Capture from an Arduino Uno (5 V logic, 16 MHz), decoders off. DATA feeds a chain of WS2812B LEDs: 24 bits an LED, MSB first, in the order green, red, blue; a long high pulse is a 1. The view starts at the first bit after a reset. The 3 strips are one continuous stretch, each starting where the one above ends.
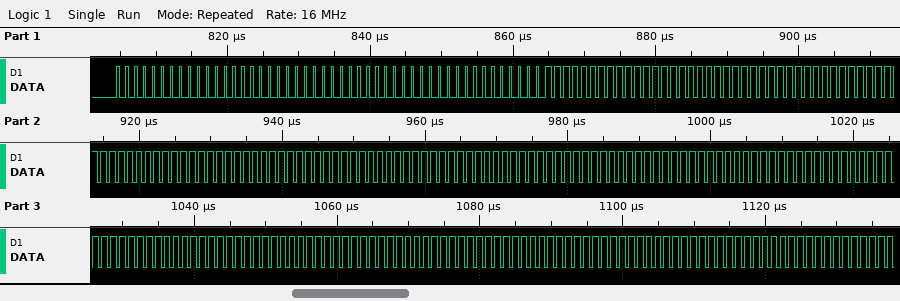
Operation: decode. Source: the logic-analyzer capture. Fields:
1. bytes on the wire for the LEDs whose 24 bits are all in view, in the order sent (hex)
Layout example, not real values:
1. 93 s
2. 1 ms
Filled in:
1. 00 00 00 00 00 00 FF FF FF FF FF FF FF FF FF FF FF FF FF FF FF FF FF FF FF FF FF FF FF FF FF FF FF
